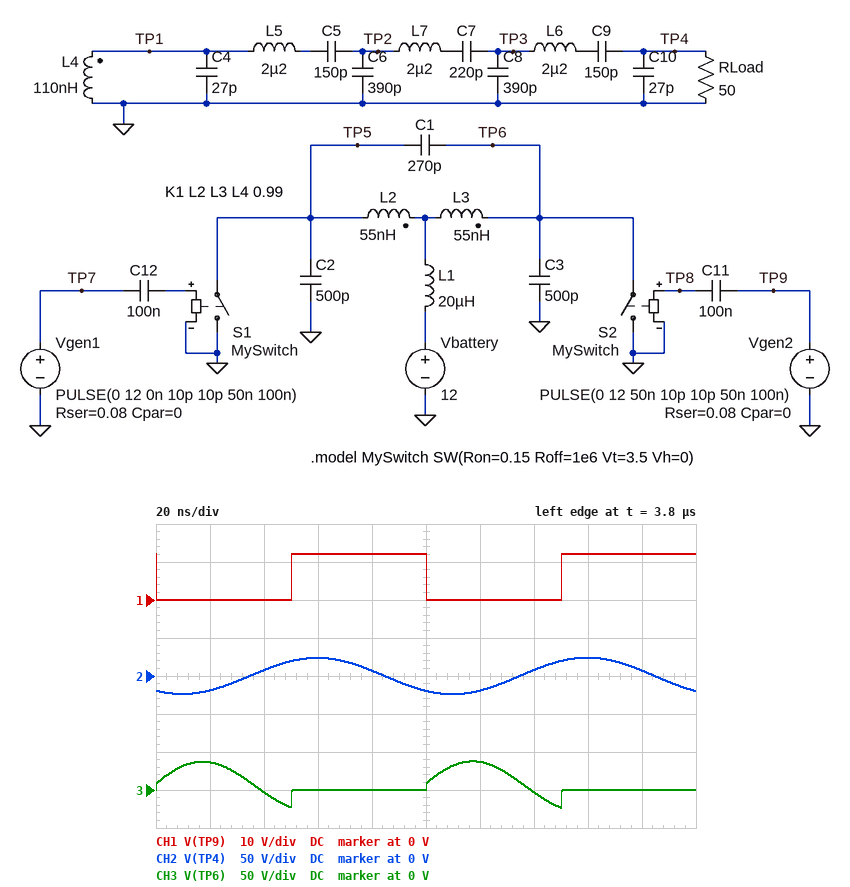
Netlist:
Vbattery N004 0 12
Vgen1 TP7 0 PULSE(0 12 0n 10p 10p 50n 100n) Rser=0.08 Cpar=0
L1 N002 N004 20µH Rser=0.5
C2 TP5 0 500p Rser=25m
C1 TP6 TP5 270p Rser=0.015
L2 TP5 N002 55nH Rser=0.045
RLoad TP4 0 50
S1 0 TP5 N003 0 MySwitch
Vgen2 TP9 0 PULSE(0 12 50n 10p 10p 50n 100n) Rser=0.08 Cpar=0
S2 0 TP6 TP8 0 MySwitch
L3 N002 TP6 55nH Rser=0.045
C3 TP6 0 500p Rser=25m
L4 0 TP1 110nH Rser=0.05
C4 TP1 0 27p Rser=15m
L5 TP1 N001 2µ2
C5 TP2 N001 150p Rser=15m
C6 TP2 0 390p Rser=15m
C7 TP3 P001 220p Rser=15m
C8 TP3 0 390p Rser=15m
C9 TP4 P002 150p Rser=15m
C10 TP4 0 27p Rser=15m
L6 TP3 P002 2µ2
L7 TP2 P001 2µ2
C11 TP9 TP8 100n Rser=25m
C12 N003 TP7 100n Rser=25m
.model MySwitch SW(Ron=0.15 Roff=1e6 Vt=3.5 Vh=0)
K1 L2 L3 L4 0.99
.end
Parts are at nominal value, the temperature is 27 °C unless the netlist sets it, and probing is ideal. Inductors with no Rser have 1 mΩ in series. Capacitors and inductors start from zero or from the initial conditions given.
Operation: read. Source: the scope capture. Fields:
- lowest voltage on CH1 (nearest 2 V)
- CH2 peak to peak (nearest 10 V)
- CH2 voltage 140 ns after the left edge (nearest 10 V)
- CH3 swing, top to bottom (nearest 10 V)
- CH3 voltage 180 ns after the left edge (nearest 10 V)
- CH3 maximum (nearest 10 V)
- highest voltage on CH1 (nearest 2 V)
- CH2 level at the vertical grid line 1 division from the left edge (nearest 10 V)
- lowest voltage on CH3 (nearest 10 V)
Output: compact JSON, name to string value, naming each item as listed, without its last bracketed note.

{"lowest voltage on CH1": "0 V", "CH2 peak to peak": "50 V", "CH2 voltage 140 ns after the left edge": "10 V", "CH3 swing, top to bottom": "60 V", "CH3 voltage 180 ns after the left edge": "0 V", "CH3 maximum": "40 V", "highest voltage on CH1": "12 V", "CH2 level at the vertical grid line 1 division from the left edge": "-20 V", "lowest voltage on CH3": "-20 V"}
